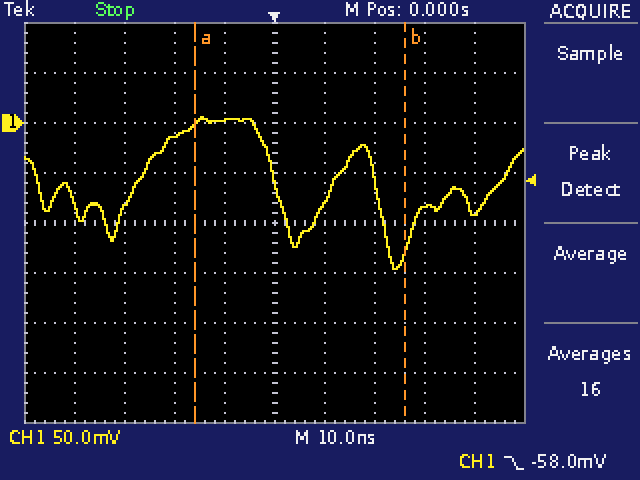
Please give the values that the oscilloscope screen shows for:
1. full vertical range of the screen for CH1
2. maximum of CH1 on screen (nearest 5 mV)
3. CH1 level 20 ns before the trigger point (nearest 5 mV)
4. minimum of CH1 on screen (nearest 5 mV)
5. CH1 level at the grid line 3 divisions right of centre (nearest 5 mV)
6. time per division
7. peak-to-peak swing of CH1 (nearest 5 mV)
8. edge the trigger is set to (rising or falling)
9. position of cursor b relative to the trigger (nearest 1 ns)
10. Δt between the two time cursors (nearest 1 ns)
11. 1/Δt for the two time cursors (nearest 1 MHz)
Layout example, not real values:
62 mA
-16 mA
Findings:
400 mV
5 mV
-15 mV
-145 mV
-85 mV
10 ns
150 mV
falling
+26 ns
42 ns
24 MHz
